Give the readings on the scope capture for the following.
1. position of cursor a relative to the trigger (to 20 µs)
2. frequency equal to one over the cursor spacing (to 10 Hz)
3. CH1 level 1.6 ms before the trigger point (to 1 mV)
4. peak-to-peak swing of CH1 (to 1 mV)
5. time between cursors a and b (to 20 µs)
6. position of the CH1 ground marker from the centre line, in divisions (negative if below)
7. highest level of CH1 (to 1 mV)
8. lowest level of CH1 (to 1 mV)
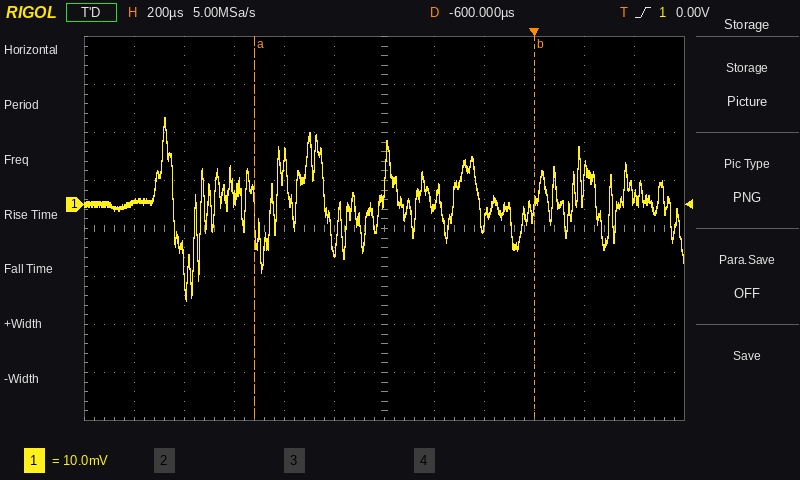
-1.12 ms
890 Hz
1 mV
38 mV
1.12 ms
+0.5 div
18 mV
-20 mV
